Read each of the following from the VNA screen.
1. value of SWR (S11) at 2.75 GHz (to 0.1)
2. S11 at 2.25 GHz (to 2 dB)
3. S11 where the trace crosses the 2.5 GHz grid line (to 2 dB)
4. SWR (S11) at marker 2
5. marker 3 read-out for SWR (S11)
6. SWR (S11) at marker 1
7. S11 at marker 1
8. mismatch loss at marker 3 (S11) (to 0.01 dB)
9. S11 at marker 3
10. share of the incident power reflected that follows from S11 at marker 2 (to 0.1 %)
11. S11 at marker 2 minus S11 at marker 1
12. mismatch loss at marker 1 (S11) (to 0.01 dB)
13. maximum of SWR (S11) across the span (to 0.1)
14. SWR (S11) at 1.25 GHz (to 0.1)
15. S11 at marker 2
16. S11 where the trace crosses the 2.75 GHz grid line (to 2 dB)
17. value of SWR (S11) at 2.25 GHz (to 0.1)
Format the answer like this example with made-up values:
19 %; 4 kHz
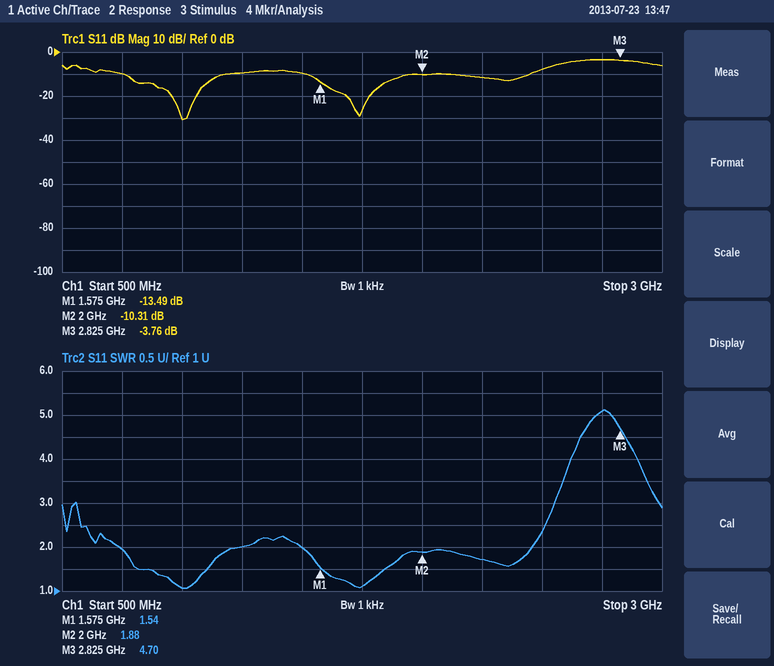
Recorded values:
5.1; -12 dB; -8 dB; 1.88; 4.70; 1.54; -13.49 dB; 2.37 dB; -3.76 dB; 9.3 %; 3.18 dB; 0.20 dB; 5.1; 2.0; -10.31 dB; -4 dB; 1.7
